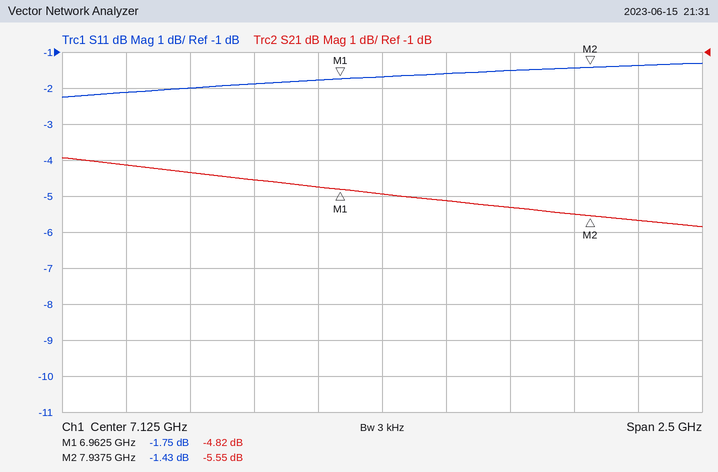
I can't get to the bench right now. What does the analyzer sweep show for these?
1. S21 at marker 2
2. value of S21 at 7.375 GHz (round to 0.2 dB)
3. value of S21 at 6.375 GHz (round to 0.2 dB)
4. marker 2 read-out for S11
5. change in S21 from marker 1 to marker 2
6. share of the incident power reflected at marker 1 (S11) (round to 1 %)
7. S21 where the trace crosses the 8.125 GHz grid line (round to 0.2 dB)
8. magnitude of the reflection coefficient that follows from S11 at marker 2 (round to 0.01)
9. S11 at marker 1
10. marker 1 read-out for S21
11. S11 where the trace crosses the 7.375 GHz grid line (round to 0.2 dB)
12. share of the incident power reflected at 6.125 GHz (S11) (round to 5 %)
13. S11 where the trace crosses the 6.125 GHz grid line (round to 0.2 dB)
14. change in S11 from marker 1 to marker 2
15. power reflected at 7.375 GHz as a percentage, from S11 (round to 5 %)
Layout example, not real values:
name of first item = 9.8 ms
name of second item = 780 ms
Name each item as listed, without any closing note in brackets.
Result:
S21 at marker 2 = -5.55 dB
value of S21 at 7.375 GHz = -5.2 dB
value of S21 at 6.375 GHz = -4.4 dB
marker 2 read-out for S11 = -1.43 dB
change in S21 from marker 1 to marker 2 = -0.73 dB
share of the incident power reflected at marker 1 (S11) = 67 %
S21 where the trace crosses the 8.125 GHz grid line = -5.6 dB
magnitude of the reflection coefficient that follows from S11 at marker 2 = 0.85
S11 at marker 1 = -1.75 dB
marker 1 read-out for S21 = -4.82 dB
S11 where the trace crosses the 7.375 GHz grid line = -1.6 dB
share of the incident power reflected at 6.125 GHz (S11) = 60 %
S11 where the trace crosses the 6.125 GHz grid line = -2.2 dB
change in S11 from marker 1 to marker 2 = 0.32 dB
power reflected at 7.375 GHz as a percentage, from S11 = 70 %
